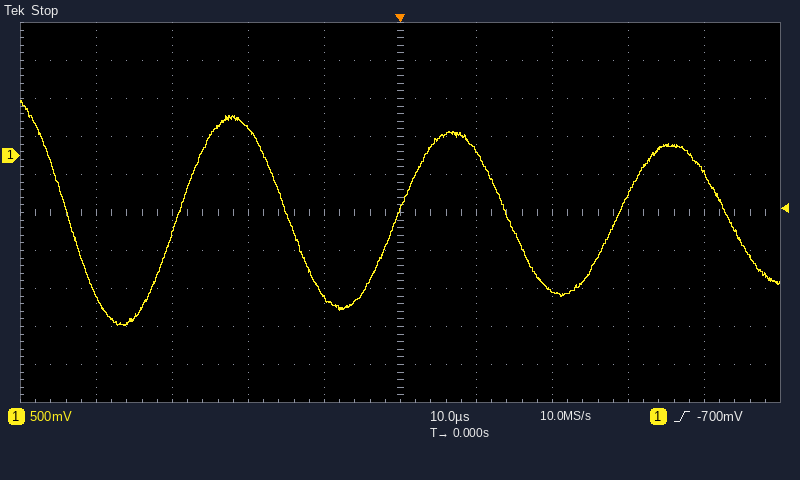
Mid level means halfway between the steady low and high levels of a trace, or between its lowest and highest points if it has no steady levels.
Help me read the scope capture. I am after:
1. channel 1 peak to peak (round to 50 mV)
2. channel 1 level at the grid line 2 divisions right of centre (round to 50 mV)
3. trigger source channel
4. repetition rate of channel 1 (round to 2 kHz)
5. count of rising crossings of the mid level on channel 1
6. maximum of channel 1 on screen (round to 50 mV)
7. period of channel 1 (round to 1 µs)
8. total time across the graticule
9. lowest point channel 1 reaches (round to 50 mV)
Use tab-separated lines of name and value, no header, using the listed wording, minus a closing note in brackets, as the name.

channel 1 peak to peak	2.95 V
channel 1 level at the grid line 2 divisions right of centre	-1.80 V
trigger source channel	channel 1
repetition rate of channel 1	34 kHz
count of rising crossings of the mid level on channel 1	3
maximum of channel 1 on screen	700 mV
period of channel 1	29 µs
total time across the graticule	100 µs
lowest point channel 1 reaches	-2.25 V
